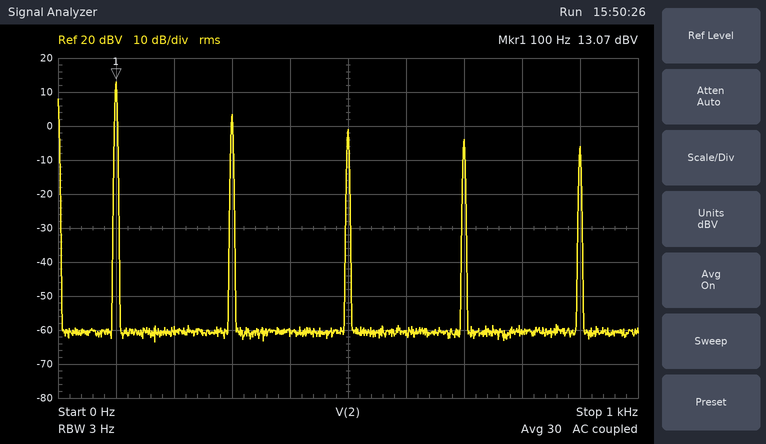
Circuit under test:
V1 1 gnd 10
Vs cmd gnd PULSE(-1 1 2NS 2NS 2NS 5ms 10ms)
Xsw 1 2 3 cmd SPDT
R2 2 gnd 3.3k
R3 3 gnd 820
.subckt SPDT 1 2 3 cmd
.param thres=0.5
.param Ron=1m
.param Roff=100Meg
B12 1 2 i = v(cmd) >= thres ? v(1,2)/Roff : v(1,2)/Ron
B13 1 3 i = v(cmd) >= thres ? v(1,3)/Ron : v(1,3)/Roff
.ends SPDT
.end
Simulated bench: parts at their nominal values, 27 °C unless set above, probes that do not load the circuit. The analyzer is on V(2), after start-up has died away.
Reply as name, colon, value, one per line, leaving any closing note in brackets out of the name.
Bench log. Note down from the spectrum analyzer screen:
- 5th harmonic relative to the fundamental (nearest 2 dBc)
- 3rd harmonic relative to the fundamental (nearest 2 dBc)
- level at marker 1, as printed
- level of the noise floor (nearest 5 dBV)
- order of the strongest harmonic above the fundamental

5th harmonic relative to the fundamental: -14 dBc
3rd harmonic relative to the fundamental: -10 dBc
level at marker 1, as printed: 13.07 dBV
level of the noise floor: -60 dBV
order of the strongest harmonic above the fundamental: 3
